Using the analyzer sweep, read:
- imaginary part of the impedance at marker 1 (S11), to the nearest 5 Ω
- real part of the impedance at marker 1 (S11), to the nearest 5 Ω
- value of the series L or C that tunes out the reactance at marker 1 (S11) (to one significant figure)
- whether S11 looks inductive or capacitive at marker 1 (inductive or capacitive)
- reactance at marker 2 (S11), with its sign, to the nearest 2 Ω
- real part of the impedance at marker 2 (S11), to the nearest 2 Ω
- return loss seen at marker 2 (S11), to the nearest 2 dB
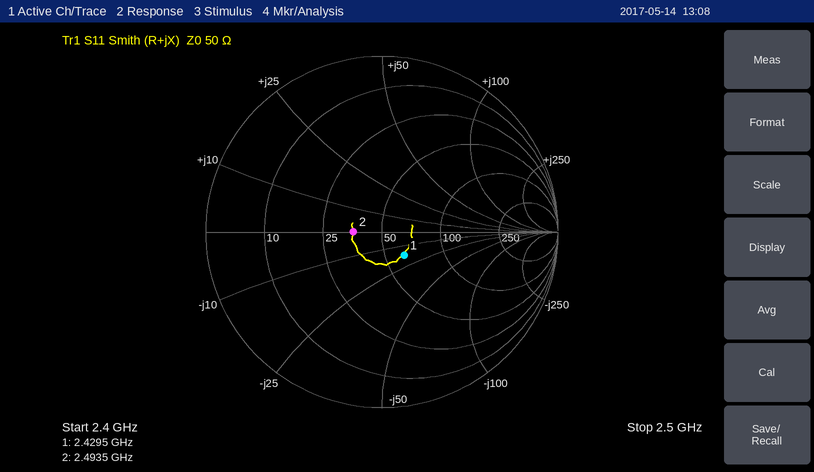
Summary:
-15 Ω
60 Ω
1 nH
capacitive
0 Ω
36 Ω
16 dB
